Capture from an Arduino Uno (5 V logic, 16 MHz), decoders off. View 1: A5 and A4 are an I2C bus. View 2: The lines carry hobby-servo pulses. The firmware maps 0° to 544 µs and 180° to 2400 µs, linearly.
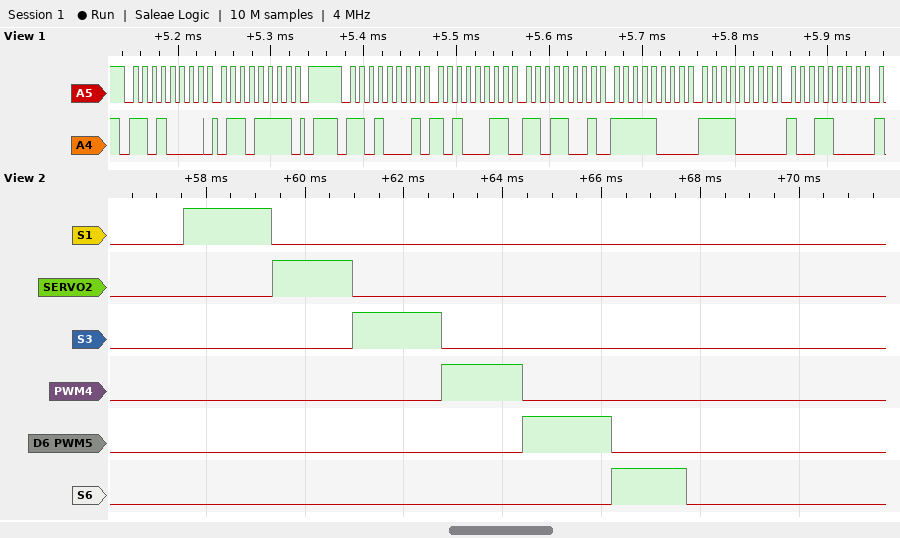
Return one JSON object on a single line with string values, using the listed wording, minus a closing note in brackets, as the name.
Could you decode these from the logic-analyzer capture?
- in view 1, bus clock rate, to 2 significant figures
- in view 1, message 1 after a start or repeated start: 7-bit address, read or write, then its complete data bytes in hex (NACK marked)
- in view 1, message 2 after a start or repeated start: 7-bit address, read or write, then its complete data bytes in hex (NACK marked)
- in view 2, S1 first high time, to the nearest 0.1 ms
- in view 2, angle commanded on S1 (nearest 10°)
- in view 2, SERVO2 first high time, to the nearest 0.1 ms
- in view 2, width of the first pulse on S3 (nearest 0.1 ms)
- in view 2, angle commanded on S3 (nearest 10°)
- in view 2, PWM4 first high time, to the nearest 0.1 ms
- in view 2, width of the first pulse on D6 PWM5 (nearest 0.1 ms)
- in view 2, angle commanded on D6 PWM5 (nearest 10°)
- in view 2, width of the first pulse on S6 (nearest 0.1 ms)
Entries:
{"in view 1, bus clock rate, to 2 significant figures": "100 kHz", "in view 1, message 1 after a start or repeated start: 7-bit address, read or write, then its complete data bytes in hex": "0x68 write: 6F", "in view 1, message 2 after a start or repeated start: 7-bit address, read or write, then its complete data bytes in hex": "0x68 read: A3 D9 F8 F0 98", "in view 2, S1 first high time, to the nearest 0.1 ms": "1.8 ms", "in view 2, angle commanded on S1": "120°", "in view 2, SERVO2 first high time, to the nearest 0.1 ms": "1.6 ms", "in view 2, width of the first pulse on S3": "1.8 ms", "in view 2, angle commanded on S3": "120°", "in view 2, PWM4 first high time, to the nearest 0.1 ms": "1.6 ms", "in view 2, width of the first pulse on D6 PWM5": "1.8 ms", "in view 2, angle commanded on D6 PWM5": "120°", "in view 2, width of the first pulse on S6": "1.5 ms"}
